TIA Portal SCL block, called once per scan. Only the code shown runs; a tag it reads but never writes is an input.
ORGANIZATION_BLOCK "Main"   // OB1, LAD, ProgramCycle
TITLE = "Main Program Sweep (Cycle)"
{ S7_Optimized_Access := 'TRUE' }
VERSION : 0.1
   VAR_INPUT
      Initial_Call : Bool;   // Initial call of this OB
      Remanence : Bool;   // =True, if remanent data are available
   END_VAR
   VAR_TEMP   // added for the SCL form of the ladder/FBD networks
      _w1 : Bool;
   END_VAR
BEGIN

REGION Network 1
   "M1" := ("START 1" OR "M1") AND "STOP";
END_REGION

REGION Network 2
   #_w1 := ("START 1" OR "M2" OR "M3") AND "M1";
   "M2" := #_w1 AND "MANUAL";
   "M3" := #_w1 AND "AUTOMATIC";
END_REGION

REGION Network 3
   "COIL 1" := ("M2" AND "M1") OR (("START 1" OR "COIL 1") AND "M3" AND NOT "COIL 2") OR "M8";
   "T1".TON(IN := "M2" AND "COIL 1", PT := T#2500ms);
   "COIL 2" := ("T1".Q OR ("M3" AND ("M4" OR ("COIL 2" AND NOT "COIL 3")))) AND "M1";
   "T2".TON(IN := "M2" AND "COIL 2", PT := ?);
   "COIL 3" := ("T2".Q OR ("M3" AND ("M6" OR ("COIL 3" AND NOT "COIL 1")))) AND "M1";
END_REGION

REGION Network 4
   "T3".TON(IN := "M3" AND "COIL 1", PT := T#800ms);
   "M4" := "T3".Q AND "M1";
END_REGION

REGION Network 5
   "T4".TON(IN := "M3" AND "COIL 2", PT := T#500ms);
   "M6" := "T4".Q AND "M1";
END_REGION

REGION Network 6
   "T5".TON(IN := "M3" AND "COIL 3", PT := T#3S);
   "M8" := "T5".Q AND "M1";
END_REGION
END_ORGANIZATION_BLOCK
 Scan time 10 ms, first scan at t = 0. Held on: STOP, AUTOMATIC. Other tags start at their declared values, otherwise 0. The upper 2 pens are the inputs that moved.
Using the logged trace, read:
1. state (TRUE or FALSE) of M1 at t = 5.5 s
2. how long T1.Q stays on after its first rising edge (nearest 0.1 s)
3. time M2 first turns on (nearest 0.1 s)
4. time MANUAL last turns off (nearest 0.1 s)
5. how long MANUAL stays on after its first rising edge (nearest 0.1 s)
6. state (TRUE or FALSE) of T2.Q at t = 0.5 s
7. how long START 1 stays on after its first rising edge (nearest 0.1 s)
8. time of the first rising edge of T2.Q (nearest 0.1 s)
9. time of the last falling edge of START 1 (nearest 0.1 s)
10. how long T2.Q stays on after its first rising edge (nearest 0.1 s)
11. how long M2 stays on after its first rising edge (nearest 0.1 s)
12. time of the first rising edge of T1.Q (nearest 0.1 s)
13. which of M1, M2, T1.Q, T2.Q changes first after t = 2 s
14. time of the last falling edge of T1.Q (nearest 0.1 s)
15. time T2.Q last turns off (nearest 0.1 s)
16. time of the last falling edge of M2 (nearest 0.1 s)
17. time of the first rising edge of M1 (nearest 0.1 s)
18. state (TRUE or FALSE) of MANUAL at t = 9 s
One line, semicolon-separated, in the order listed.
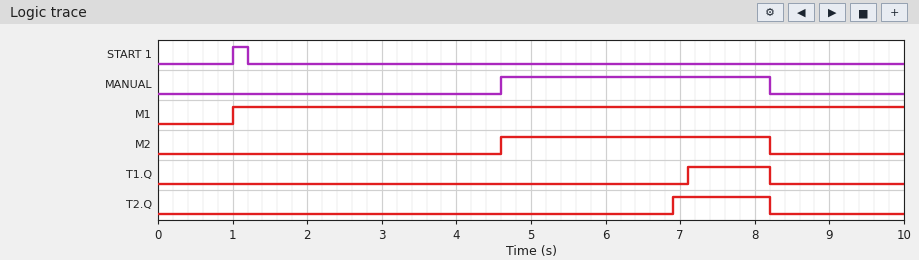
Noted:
TRUE; 1.1 s; 4.6 s; 8.2 s; 3.6 s; FALSE; 0.2 s; 6.9 s; 1.2 s; 1.3 s; 3.6 s; 7.1 s; M2; 8.2 s; 8.2 s; 8.2 s; 1.0 s; FALSE
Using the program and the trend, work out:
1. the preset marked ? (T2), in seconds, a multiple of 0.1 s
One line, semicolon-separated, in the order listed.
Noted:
1.5 s
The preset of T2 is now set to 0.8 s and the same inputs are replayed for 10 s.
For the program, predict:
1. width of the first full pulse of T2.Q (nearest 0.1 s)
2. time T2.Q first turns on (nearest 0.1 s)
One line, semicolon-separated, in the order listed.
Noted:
2.0 s; 6.2 s
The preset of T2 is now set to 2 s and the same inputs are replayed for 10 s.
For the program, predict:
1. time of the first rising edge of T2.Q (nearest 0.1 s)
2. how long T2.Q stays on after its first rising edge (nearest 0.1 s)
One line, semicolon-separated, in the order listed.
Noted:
7.4 s; 0.8 s
